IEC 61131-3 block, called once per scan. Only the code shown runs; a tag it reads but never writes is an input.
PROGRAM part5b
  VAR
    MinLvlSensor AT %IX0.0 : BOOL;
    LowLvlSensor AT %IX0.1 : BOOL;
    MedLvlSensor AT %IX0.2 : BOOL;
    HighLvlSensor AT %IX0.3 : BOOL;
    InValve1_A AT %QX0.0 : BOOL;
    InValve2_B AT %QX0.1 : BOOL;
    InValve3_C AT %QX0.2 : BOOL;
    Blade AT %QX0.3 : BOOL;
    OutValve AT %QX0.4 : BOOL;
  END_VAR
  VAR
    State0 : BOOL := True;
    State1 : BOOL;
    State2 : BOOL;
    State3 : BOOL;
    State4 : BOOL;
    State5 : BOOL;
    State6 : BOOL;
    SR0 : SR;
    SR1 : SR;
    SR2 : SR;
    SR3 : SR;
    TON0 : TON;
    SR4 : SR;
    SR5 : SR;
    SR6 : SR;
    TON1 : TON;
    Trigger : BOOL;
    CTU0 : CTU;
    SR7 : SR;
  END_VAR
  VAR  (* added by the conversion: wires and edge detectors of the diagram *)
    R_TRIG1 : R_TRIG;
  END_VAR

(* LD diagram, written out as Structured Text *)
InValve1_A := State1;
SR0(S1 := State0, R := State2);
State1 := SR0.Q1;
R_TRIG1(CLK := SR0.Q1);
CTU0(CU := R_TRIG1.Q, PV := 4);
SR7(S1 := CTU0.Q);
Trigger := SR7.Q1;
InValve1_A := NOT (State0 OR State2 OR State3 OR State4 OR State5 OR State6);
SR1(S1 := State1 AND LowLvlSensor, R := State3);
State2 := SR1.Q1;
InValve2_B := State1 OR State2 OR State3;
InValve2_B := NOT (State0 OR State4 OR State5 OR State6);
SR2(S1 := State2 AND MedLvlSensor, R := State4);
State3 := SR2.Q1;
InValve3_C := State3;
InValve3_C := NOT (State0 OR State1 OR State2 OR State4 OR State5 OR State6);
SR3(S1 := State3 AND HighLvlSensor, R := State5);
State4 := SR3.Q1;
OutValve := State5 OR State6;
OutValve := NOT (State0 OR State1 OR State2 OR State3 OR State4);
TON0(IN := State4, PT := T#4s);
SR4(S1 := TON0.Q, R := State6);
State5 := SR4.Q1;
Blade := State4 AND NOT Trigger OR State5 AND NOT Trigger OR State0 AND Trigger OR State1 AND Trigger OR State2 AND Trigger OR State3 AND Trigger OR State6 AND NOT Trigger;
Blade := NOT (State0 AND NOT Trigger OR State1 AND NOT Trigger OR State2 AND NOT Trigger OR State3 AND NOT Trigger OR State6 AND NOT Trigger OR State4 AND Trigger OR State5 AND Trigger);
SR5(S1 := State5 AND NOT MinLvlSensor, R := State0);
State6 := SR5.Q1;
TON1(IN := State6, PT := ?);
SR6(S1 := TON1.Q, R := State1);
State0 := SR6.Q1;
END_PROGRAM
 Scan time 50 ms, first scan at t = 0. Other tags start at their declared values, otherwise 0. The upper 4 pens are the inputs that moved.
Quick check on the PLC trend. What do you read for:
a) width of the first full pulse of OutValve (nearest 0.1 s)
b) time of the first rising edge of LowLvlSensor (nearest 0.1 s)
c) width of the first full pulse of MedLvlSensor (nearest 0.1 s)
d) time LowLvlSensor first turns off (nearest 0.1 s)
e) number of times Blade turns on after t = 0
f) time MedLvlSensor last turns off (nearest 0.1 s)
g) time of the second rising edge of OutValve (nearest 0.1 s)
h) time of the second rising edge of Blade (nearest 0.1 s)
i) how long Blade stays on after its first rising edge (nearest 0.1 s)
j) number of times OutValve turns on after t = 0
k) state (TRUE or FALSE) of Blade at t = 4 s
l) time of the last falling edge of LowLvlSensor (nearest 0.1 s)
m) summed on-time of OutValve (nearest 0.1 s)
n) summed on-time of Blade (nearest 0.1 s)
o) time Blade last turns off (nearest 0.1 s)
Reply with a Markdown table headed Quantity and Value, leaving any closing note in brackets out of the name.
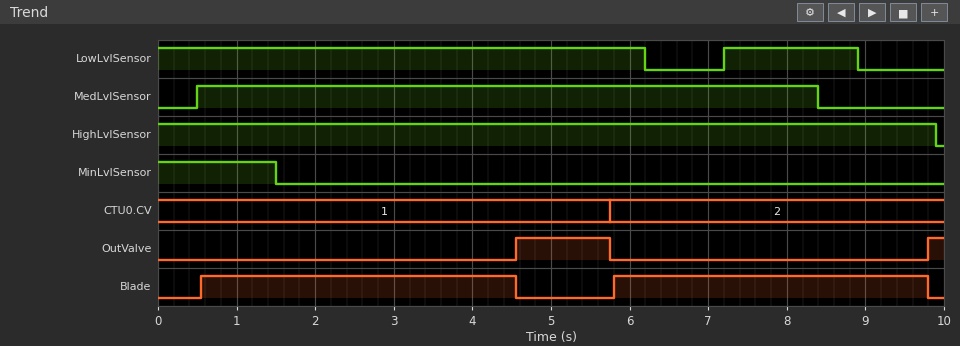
| Quantity | Value |
|---|---|
| width of the first full pulse of OutValve | 1.2 s |
| time of the first rising edge of LowLvlSensor | 7.2 s |
| width of the first full pulse of MedLvlSensor | 7.9 s |
| time LowLvlSensor first turns off | 6.2 s |
| number of times Blade turns on after t = 0 | 2 |
| time MedLvlSensor last turns off | 8.4 s |
| time of the second rising edge of OutValve | 9.8 s |
| time of the second rising edge of Blade | 5.8 s |
| how long Blade stays on after its first rising edge | 4.0 s |
| number of times OutValve turns on after t = 0 | 2 |
| state (TRUE or FALSE) of Blade at t = 4 s | TRUE |
| time of the last falling edge of LowLvlSensor | 8.9 s |
| summed on-time of OutValve | 1.4 s |
| summed on-time of Blade | 8.0 s |
| time Blade last turns off | 9.8 s |
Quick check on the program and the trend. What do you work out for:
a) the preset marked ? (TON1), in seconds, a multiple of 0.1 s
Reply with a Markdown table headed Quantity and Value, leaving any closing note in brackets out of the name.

| Quantity | Value |
|---|---|
| the preset marked ? (TON1), in seconds, a multiple of 0.1 s | 1.2 s |
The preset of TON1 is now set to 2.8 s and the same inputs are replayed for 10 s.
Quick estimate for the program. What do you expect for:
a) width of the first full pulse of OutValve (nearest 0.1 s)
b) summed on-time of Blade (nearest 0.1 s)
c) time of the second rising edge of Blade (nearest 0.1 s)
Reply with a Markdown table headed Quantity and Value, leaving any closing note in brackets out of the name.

| Quantity | Value |
|---|---|
| width of the first full pulse of OutValve | 2.8 s |
| summed on-time of Blade | 6.6 s |
| time of the second rising edge of Blade | 7.4 s |
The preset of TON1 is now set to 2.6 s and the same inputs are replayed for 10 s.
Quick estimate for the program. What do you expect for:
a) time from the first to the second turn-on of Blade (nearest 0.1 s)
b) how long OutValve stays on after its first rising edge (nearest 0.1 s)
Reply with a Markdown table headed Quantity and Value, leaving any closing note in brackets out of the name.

| Quantity | Value |
|---|---|
| time from the first to the second turn-on of Blade | 6.7 s |
| how long OutValve stays on after its first rising edge | 2.6 s |
